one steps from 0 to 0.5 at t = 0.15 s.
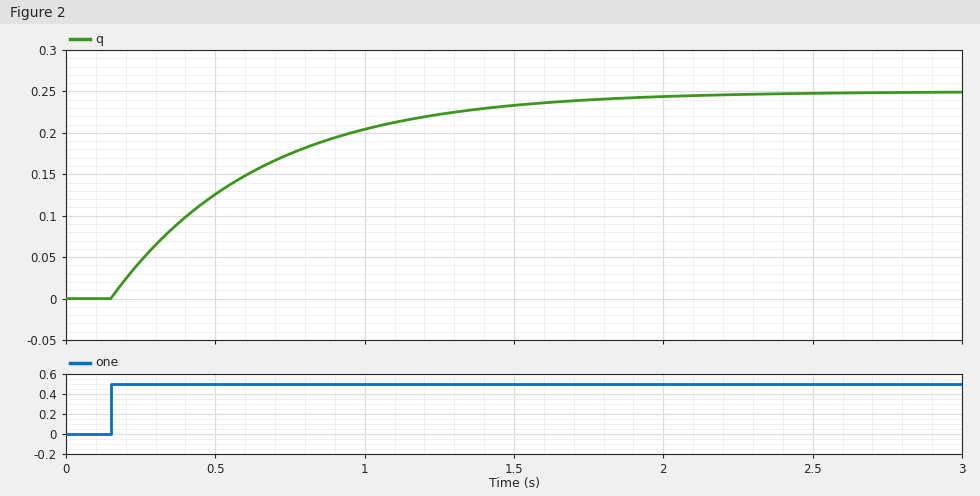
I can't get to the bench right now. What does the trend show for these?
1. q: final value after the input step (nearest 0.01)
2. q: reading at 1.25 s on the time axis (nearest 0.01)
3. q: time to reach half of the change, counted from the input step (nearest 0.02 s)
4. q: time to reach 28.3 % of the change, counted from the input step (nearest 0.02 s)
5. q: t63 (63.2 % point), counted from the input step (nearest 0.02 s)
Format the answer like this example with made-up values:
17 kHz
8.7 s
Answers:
0.25
0.22
0.34 s
0.16 s
0.50 s
